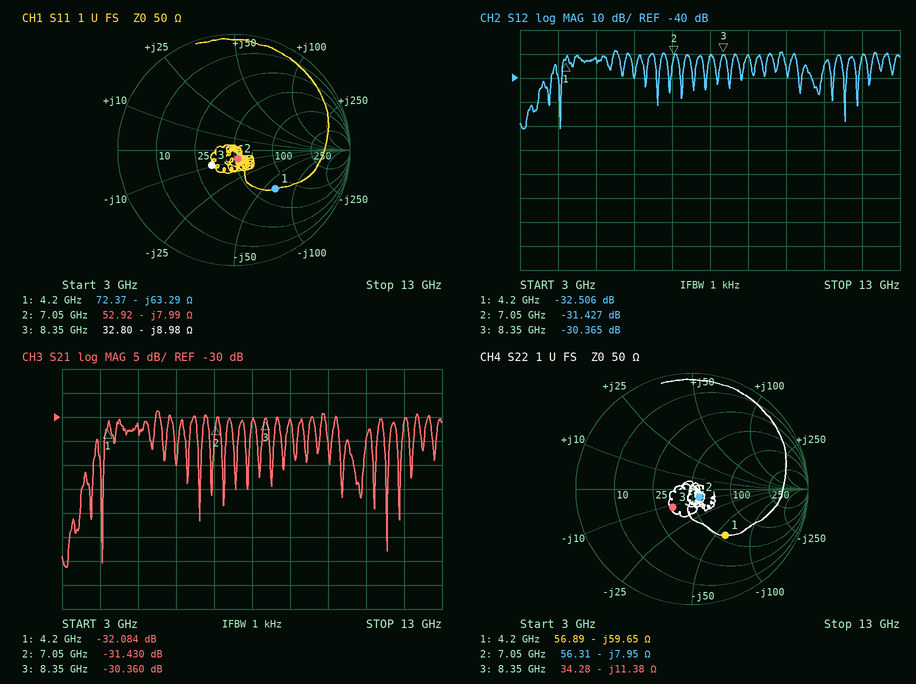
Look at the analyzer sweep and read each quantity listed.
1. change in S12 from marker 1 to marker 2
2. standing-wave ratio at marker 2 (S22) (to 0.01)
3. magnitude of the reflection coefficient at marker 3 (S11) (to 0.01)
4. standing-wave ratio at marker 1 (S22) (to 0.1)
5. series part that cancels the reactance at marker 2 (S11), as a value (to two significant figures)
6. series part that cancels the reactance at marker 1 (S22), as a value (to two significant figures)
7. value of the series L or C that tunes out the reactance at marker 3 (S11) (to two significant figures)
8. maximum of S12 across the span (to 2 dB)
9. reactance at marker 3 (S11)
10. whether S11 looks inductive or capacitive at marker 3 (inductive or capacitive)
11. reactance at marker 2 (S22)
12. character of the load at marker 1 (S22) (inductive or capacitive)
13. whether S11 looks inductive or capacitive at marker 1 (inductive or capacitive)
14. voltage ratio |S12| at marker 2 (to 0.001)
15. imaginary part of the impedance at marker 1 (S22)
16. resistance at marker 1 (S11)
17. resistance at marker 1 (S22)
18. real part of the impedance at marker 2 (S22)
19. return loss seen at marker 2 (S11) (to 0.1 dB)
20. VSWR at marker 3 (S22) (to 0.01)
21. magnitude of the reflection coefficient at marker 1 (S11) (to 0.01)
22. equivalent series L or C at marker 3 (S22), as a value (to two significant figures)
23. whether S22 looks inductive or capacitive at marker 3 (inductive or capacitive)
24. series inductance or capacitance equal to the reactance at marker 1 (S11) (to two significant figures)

1.079 dB
1.21
0.23
2.9
180 pH
2.3 nH
170 pH
-28 dB
-8.98 Ω
capacitive
-7.95 Ω
capacitive
capacitive
0.027
-59.65 Ω
72.37 Ω
56.89 Ω
56.31 Ω
21.7 dB
1.59
0.49
1.7 pF
capacitive
600 fF
